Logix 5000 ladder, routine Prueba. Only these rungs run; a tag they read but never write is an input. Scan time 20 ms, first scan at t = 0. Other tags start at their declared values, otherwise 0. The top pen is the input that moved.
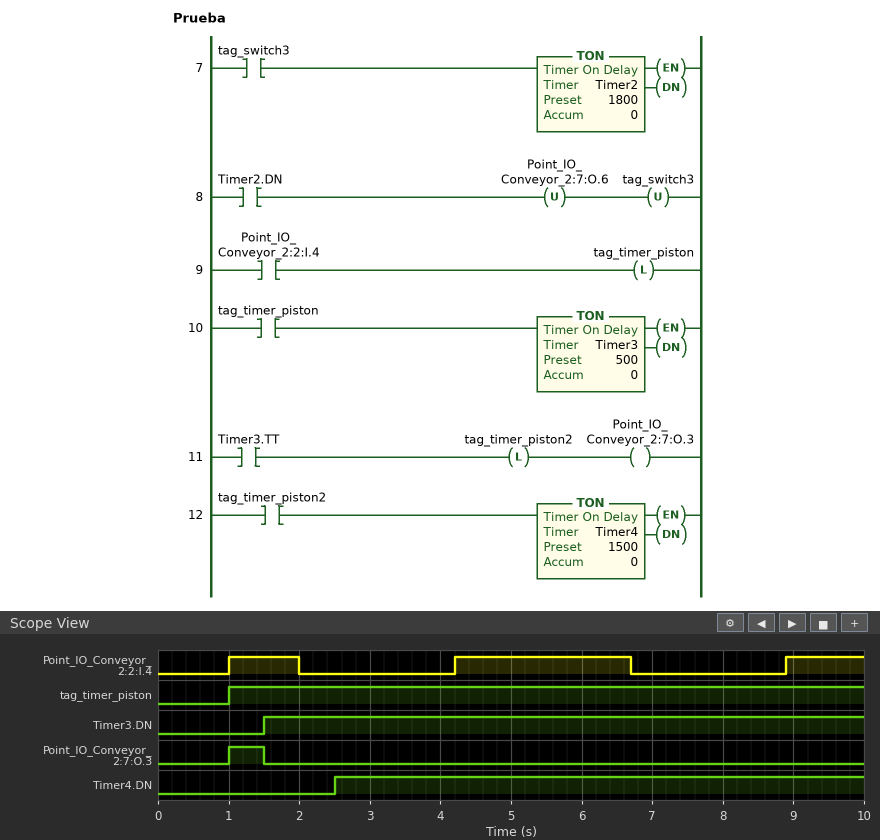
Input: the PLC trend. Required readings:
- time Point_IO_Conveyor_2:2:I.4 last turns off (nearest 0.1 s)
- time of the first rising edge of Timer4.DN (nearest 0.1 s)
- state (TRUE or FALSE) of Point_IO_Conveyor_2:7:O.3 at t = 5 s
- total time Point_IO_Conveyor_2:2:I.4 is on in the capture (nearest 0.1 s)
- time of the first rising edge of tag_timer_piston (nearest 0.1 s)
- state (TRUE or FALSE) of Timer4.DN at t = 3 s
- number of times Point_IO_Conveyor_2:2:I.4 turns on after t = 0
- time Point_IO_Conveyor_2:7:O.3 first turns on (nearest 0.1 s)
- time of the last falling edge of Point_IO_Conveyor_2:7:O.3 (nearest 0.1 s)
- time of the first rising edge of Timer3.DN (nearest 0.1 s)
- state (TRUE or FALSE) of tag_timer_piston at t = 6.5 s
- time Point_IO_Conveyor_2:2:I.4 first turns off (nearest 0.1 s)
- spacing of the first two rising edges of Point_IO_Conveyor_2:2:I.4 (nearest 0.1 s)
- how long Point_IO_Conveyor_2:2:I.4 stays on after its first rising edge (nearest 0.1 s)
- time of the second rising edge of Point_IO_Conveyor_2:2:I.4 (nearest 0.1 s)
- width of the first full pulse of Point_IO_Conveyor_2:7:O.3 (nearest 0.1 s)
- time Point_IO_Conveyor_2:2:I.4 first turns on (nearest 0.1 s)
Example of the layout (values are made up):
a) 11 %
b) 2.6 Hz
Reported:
a) 6.7 s
b) 2.5 s
c) FALSE
d) 4.6 s
e) 1.0 s
f) TRUE
g) 3
h) 1.0 s
i) 1.5 s
j) 1.5 s
k) TRUE
l) 2.0 s
m) 3.2 s
n) 1.0 s
o) 4.2 s
p) 0.5 s
q) 1.0 s
